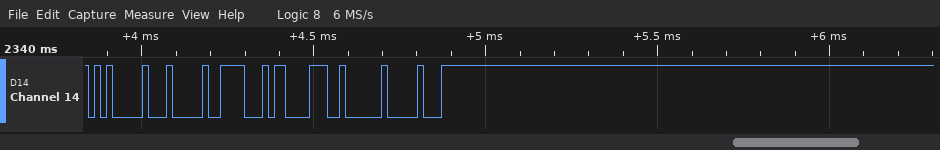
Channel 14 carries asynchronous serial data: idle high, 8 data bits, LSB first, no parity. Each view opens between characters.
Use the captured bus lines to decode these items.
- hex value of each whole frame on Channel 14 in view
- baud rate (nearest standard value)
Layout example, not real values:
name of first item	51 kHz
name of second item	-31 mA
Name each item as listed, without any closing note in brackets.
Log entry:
hex value of each whole frame on Channel 14 in view	05, 04, 1E, C3, 02, 10
baud rate	57600 baud
